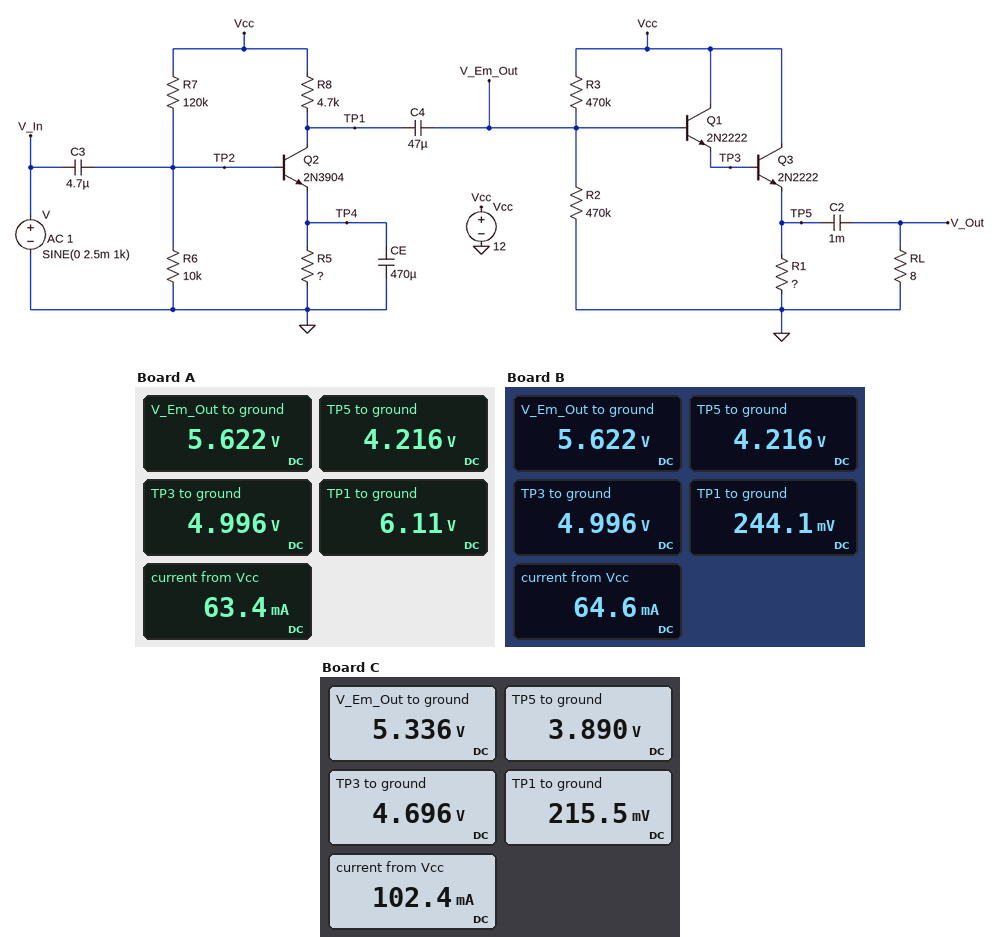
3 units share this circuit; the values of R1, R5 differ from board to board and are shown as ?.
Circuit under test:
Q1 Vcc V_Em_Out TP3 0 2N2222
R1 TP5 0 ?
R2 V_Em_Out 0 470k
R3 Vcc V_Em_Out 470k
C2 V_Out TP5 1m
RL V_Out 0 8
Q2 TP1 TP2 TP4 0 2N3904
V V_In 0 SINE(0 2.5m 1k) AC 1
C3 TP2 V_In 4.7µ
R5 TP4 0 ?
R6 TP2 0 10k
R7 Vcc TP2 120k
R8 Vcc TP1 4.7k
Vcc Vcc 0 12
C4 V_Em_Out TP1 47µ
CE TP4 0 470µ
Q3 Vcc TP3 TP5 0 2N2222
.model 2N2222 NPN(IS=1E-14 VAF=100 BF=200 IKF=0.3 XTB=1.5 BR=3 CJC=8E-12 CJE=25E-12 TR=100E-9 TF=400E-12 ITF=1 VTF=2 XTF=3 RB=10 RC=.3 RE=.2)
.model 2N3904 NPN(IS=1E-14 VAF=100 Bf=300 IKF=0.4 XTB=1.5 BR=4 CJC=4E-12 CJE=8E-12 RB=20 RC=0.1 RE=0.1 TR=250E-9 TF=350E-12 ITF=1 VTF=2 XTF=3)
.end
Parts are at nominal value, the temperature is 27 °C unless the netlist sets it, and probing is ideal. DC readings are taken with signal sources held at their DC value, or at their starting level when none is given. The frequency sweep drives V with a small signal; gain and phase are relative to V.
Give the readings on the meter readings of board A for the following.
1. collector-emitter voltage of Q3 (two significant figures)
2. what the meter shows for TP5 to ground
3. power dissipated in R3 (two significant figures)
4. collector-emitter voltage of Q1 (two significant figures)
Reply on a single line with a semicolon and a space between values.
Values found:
7.8 V; 4.216 V; 87 µW; 7.0 V
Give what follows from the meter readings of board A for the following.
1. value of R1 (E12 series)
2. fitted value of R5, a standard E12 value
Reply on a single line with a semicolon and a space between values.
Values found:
68 Ω; 180 Ω
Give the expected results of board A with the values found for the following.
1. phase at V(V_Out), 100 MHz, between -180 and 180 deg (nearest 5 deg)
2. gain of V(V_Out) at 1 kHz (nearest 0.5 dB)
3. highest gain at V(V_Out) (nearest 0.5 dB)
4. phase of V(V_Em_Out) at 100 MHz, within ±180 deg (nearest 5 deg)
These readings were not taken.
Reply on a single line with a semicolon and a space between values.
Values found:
55 deg; 45.0 dB; 45.0 dB; 80 deg
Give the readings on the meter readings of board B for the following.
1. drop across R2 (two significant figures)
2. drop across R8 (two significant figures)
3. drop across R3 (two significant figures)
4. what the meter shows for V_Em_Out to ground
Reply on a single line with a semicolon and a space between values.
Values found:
5.6 V; 12 V; 6.4 V; 5.622 V
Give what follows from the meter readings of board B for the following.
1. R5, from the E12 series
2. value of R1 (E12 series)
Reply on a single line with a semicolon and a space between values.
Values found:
47 Ω; 68 Ω
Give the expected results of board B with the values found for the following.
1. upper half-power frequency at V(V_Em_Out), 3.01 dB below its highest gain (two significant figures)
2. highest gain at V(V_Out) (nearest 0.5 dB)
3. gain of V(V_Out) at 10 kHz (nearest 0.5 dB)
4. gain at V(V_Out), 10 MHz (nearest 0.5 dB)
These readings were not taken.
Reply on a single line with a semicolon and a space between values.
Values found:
430 kHz; 34.0 dB; 34.0 dB; 6.0 dB
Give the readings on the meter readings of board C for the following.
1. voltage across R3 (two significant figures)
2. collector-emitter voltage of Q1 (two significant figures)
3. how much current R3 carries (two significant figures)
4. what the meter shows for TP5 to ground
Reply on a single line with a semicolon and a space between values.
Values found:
6.7 V; 7.3 V; 14 µA; 3.890 V
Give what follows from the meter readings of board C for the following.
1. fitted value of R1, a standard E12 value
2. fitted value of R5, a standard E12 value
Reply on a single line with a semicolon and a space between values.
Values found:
39 Ω; 39 Ω
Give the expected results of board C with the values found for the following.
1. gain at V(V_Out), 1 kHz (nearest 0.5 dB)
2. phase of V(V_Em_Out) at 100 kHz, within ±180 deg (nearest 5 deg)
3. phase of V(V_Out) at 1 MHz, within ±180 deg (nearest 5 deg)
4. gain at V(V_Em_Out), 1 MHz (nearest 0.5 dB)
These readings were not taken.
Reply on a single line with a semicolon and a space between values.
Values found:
31.0 dB; 165 deg; 110 deg; 24.5 dB
